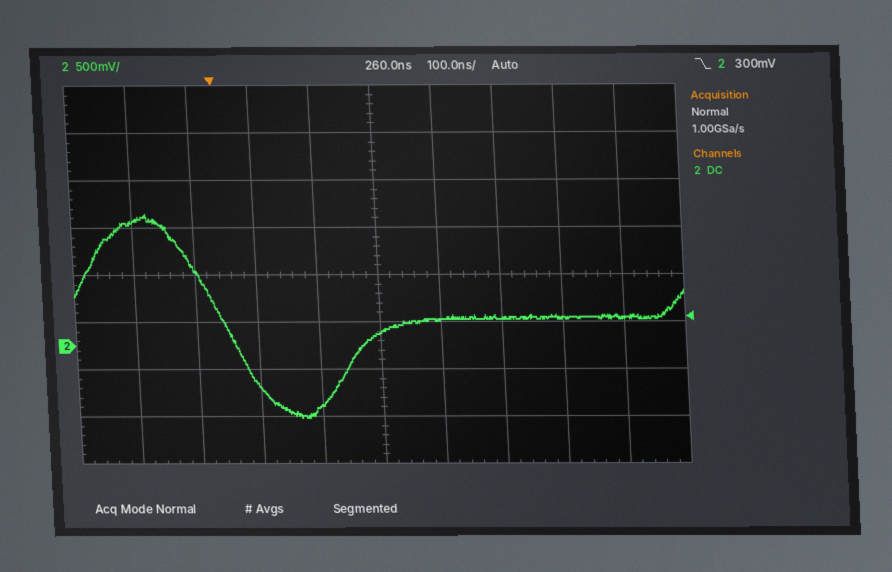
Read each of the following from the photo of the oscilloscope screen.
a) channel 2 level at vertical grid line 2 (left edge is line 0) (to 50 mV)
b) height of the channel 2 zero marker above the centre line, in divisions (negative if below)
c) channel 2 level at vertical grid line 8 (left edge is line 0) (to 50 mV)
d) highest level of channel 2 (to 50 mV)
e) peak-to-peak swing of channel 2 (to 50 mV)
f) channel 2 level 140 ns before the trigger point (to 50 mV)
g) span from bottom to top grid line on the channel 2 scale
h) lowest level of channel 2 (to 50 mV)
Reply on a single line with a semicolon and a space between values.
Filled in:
800 mV; -1.5 div; 300 mV; 1.40 V; 2.15 V; 1.30 V; 4 V; -750 mV
